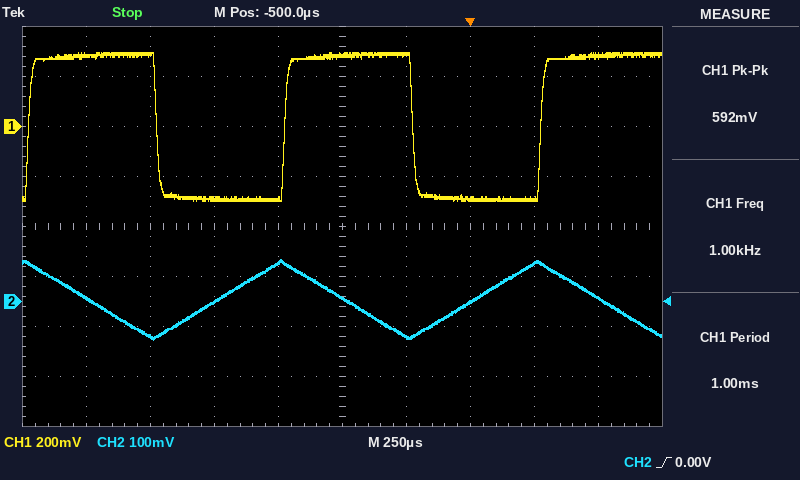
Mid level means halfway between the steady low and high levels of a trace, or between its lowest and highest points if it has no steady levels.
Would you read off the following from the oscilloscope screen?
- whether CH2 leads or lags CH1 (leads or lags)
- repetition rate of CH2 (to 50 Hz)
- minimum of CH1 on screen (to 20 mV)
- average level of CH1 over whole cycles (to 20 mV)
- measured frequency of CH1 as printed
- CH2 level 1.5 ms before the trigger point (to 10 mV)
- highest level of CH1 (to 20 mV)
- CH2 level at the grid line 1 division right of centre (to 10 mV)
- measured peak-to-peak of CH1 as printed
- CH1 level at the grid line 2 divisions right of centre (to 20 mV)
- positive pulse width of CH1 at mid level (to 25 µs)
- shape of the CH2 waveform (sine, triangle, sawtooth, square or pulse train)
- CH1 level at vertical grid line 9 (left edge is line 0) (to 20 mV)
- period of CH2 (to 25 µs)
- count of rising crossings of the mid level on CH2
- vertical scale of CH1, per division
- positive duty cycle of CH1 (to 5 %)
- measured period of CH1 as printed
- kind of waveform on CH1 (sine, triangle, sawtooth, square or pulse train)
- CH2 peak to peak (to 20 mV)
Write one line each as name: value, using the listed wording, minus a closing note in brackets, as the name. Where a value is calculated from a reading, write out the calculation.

whether CH2 leads or lags CH1: leads
repetition rate of CH2: 1 / 1.000 ms ≈ 1.00 kHz
minimum of CH1 on screen: -300 mV
average level of CH1 over whole cycles: -300 mV + 0.5 × (300 mV − (-300 mV)) ≈ 0 mV
measured frequency of CH1 as printed: 1.00 kHz
CH2 level 1.5 ms before the trigger point: 10 mV
highest level of CH1: 300 mV
CH2 level at the grid line 1 division right of centre: -70 mV
measured peak-to-peak of CH1 as printed: 592 mV
CH1 level at the grid line 2 divisions right of centre: -280 mV
positive pulse width of CH1 at mid level: 500 µs
shape of the CH2 waveform: triangle
CH1 level at vertical grid line 9 (left edge is line 0): 280 mV
period of CH2: 1.000 ms
count of rising crossings of the mid level on CH2: 2
vertical scale of CH1, per division: 200 mV
positive duty cycle of CH1: 50 %
measured period of CH1 as printed: 1.00 ms
kind of waveform on CH1: square
CH2 peak to peak: 160 mV
